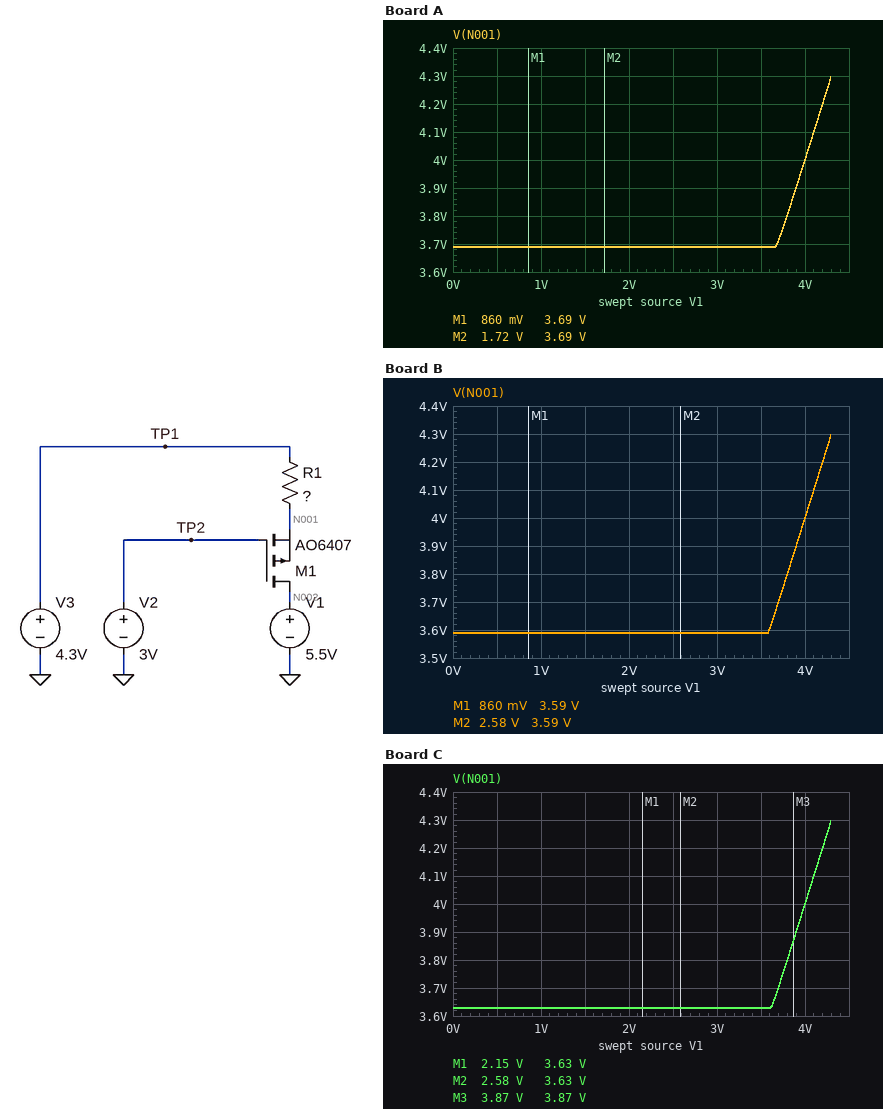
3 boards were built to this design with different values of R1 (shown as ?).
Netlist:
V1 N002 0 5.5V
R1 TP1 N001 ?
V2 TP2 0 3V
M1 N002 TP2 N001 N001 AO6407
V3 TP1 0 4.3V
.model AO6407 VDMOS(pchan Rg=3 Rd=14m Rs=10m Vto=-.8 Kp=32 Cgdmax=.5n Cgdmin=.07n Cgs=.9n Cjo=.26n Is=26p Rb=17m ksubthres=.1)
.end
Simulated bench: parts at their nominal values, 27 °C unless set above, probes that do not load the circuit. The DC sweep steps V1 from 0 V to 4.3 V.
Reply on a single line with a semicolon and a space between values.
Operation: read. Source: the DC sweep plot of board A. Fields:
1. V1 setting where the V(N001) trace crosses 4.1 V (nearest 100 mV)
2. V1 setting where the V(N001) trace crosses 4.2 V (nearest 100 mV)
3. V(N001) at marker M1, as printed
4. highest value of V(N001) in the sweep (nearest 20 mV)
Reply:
4.1 V; 4.2 V; 3.69 V; 4.30 V
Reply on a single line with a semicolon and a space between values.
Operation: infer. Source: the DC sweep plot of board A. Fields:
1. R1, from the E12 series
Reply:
47 Ω
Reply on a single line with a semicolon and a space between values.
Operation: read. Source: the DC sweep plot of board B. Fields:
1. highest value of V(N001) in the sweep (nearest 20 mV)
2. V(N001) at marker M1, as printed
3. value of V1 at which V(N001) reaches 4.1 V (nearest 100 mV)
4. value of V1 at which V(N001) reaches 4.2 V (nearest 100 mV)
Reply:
4.30 V; 3.59 V; 4.1 V; 4.2 V
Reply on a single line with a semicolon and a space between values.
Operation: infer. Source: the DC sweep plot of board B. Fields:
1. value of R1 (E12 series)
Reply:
330 Ω
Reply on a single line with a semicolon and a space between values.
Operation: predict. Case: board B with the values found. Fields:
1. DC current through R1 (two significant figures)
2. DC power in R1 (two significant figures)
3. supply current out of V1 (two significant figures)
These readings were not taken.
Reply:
3.6 mA; 4.4 mW; 3.6 mA
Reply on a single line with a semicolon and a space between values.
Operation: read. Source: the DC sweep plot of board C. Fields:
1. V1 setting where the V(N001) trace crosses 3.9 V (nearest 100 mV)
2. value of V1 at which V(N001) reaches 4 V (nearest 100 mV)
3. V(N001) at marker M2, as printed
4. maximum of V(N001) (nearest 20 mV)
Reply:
3.9 V; 4.0 V; 3.63 V; 4.30 V
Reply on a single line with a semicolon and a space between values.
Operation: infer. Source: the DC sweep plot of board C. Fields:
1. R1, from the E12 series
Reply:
150 Ω
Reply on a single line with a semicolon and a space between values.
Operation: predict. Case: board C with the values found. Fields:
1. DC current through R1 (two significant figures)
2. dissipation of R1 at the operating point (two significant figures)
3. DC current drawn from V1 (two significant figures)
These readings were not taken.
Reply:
8.0 mA; 9.6 mW; 8.0 mA
